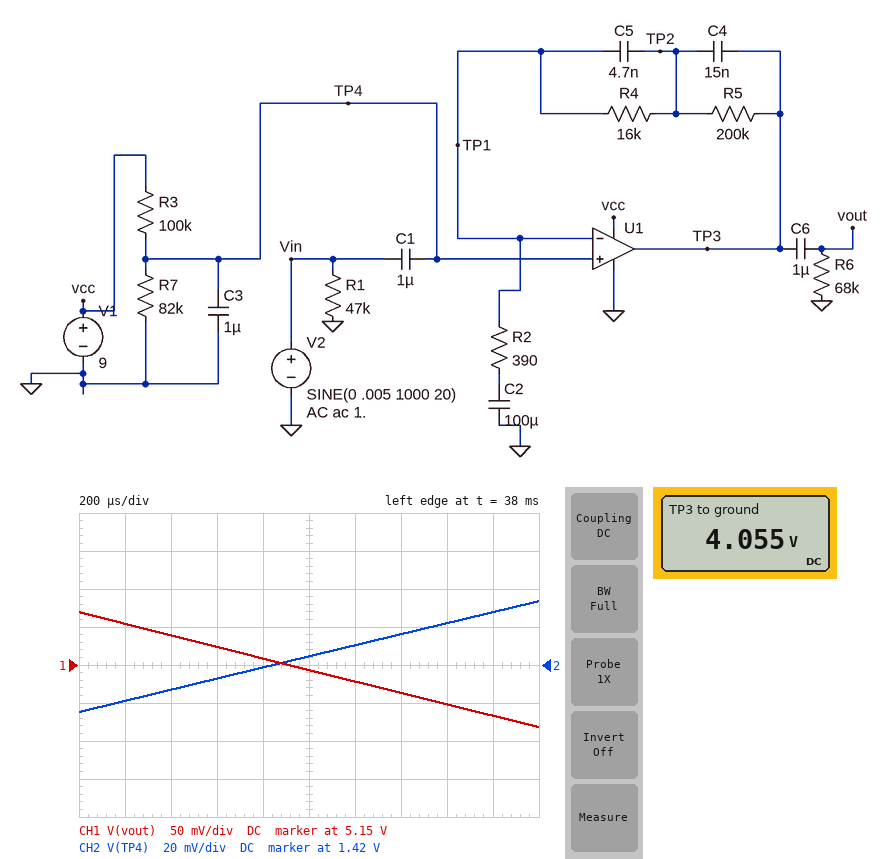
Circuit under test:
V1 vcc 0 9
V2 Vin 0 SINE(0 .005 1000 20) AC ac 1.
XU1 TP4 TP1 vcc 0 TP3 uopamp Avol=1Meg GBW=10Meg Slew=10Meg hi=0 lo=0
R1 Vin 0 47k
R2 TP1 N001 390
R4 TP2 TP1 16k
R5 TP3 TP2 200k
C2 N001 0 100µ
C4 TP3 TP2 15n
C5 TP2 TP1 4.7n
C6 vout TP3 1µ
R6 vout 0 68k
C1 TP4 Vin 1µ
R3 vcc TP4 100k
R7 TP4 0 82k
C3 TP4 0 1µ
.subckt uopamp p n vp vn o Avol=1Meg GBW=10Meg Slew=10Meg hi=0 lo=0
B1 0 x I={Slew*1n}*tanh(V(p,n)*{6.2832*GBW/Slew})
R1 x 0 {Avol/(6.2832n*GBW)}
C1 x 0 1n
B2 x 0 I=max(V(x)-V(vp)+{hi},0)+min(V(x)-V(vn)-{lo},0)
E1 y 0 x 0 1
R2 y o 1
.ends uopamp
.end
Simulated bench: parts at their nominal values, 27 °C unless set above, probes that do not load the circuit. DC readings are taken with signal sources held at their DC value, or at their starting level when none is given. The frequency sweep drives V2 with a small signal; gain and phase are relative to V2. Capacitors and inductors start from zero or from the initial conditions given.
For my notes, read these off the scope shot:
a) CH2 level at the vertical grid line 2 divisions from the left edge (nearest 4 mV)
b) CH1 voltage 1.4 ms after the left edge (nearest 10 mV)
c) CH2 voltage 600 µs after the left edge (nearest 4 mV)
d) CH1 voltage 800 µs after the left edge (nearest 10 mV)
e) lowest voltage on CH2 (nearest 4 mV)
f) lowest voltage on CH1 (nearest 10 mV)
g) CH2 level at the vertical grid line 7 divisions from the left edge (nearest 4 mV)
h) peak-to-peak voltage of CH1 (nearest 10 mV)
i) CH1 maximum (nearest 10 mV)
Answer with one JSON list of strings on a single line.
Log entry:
["1.408 V", "5.11 V", "1.412 V", "5.16 V", "1.396 V", "5.07 V", "1.436 V", "150 mV", "5.22 V"]
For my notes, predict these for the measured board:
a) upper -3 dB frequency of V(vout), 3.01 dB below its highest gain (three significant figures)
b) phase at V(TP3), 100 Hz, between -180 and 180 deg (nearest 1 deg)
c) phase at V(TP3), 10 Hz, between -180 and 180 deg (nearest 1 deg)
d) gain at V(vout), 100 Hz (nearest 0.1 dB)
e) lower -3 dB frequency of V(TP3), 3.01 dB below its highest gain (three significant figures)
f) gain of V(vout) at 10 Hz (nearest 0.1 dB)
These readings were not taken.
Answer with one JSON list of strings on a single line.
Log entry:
["63.0 Hz", "-51 deg", "22 deg", "42.4 dB", "4.13 Hz", "47.7 dB"]
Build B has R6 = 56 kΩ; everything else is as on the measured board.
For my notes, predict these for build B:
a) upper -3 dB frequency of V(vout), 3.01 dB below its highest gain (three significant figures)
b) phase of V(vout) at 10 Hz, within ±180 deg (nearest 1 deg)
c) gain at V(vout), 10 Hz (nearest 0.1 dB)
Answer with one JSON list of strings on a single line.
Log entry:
["63.4 Hz", "38 deg", "47.6 dB"]
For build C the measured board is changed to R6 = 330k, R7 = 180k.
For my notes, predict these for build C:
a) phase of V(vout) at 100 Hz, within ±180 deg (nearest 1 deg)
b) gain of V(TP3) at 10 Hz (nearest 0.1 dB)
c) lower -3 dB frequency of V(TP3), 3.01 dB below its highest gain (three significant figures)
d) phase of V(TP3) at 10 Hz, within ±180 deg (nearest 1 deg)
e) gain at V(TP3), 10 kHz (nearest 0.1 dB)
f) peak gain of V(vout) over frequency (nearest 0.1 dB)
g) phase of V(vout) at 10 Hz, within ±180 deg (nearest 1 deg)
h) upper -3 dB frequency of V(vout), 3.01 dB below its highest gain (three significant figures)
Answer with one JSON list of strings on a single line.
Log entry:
["-51 deg", "48.0 dB", "3.88 Hz", "19 deg", "15.0 dB", "48.2 dB", "22 deg", "61.6 Hz"]
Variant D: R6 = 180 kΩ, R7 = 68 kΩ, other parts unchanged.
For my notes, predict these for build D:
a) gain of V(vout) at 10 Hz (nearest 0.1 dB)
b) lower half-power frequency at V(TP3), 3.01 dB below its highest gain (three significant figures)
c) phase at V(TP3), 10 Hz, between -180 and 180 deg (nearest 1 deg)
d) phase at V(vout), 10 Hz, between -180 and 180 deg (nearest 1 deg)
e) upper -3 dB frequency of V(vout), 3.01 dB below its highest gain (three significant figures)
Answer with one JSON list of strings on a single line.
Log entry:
["47.8 dB", "4.24 Hz", "23 deg", "28 deg", "62.2 Hz"]
